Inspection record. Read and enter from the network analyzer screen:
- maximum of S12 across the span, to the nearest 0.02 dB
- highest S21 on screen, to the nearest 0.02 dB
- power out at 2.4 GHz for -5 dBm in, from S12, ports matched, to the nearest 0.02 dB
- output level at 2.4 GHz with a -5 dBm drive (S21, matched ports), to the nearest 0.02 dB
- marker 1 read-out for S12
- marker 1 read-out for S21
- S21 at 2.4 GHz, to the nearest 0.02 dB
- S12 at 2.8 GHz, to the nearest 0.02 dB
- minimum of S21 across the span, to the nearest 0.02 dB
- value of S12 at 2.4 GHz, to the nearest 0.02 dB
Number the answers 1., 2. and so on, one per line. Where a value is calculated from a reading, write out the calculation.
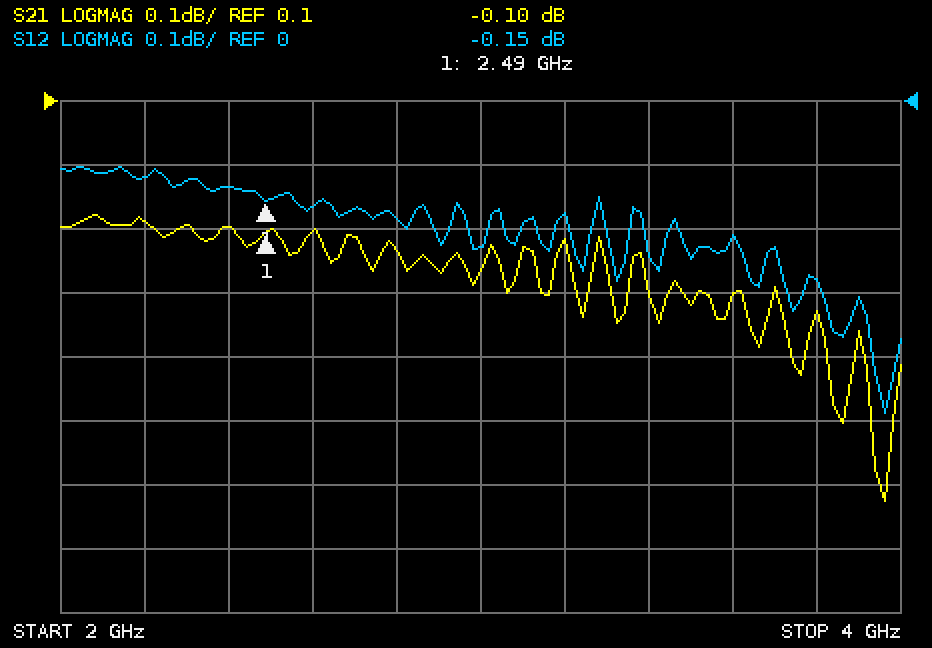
1. -0.10 dB
2. -0.08 dB
3. -5 dBm + (-0.14 dB) = -5.14 dBm
4. -5 dBm + (-0.10 dB) = -5.10 dBm
5. -0.15 dB
6. -0.10 dB
7. -0.10 dB
8. -0.18 dB
9. -0.52 dB
10. -0.14 dB
